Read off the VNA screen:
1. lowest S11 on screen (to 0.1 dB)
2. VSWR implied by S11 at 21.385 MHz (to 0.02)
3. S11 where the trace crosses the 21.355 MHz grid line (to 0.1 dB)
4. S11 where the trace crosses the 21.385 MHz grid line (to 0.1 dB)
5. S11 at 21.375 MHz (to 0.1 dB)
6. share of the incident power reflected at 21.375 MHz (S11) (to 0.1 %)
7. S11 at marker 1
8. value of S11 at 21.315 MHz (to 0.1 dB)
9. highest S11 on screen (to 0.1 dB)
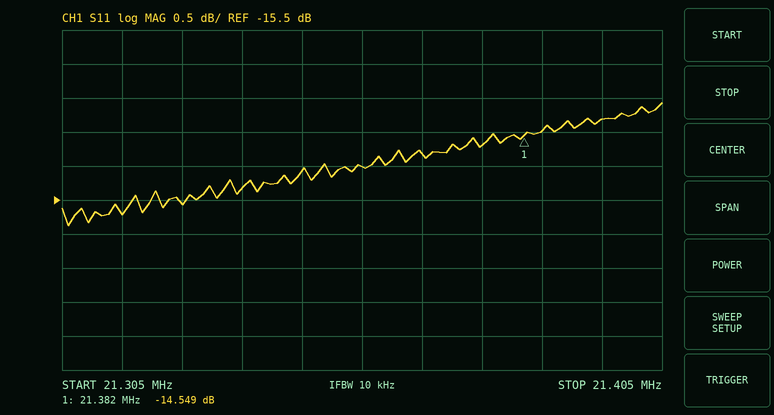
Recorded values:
-15.9 dB
1.46
-15.0 dB
-14.5 dB
-14.7 dB
3.4 %
-14.549 dB
-15.7 dB
-14.1 dB
